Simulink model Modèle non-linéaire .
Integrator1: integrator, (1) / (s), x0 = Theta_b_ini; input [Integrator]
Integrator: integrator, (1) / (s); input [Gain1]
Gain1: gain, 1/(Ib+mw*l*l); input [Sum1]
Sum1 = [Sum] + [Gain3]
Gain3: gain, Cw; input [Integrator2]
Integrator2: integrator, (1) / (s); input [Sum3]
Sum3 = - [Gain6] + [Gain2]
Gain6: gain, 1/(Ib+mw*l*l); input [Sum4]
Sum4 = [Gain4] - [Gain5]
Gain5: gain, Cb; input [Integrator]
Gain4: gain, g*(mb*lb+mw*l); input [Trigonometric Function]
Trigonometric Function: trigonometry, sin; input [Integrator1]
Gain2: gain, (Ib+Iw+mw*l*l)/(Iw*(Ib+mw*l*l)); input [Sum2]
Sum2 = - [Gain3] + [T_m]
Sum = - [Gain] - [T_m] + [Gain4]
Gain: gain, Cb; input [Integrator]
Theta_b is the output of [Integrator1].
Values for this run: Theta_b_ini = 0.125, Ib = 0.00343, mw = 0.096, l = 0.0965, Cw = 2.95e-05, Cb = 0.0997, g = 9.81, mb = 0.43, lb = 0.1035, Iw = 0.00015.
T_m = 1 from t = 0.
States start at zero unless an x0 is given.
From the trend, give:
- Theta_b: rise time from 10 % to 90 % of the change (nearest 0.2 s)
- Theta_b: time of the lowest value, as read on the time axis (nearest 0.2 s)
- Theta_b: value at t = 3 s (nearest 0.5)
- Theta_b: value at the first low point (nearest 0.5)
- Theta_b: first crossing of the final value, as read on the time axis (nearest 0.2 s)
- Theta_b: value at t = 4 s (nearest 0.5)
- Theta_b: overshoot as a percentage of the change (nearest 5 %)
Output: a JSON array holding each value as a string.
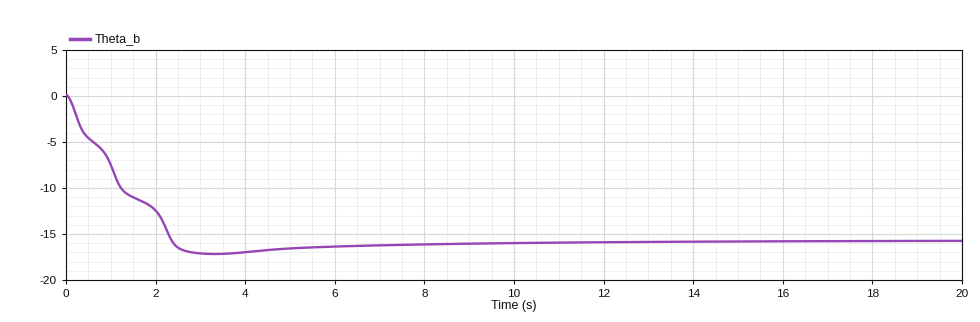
["2.0 s", "3.4 s", "-17.0", "-17.0", "2.4 s", "-17.0", "10 %"]
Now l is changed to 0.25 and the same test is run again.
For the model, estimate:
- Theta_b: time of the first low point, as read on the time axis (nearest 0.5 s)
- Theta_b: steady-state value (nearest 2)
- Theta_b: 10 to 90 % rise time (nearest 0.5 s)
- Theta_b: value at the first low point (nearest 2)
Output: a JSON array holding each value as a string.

["3.5 s", "-16", "3.0 s", "-16"]
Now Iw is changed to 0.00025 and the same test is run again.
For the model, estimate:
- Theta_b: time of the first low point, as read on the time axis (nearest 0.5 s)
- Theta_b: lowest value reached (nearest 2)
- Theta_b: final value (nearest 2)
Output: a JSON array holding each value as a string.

["6.0 s", "-30", "-28"]
